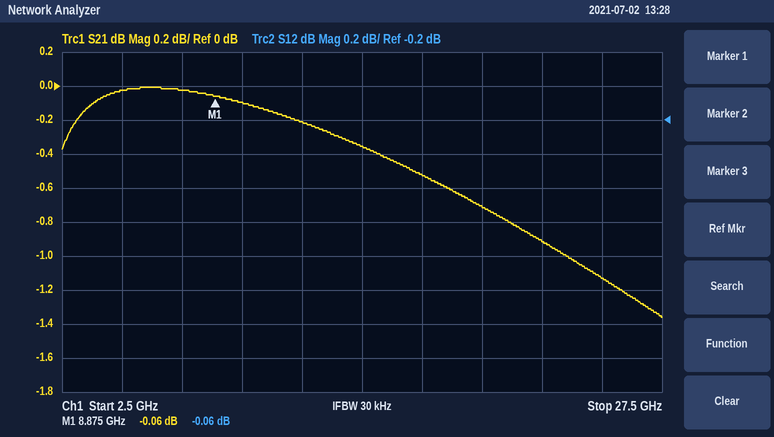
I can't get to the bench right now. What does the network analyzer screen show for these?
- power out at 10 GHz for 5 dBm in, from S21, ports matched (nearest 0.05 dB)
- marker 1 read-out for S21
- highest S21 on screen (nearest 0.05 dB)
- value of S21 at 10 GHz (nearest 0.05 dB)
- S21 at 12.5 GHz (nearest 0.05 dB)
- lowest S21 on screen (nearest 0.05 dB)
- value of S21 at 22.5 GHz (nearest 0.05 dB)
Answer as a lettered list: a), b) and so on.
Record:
a) 4.90 dBm
b) -0.06 dB
c) 0.00 dB
d) -0.10 dB
e) -0.20 dB
f) -1.35 dB
g) -0.90 dB
